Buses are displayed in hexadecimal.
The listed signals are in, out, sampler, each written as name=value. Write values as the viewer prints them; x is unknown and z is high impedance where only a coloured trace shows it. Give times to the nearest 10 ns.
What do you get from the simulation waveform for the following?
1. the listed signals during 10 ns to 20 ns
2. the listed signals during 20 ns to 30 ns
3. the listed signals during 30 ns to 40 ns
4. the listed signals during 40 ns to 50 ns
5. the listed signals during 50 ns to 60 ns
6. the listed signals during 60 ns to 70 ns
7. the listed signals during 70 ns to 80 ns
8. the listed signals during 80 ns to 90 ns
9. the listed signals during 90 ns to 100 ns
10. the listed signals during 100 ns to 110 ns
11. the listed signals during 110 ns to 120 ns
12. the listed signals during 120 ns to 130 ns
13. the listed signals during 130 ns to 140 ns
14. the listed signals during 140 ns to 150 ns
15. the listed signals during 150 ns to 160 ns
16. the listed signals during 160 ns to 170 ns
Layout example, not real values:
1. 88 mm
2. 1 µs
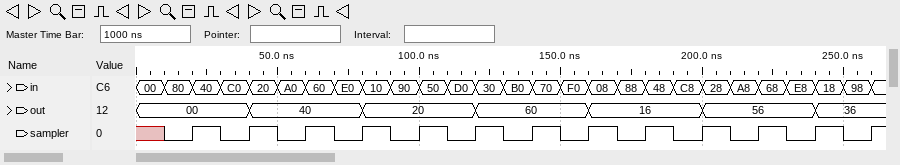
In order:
1. in=80, out=00, sampler=0
2. in=40, out=00, sampler=1
3. in=C0, out=00, sampler=0
4. in=20, out=40, sampler=1
5. in=A0, out=40, sampler=0
6. in=60, out=40, sampler=1
7. in=E0, out=40, sampler=0
8. in=10, out=20, sampler=1
9. in=90, out=20, sampler=0
10. in=50, out=20, sampler=1
11. in=D0, out=20, sampler=0
12. in=30, out=60, sampler=1
13. in=B0, out=60, sampler=0
14. in=70, out=60, sampler=1
15. in=F0, out=60, sampler=0
16. in=08, out=16, sampler=1
